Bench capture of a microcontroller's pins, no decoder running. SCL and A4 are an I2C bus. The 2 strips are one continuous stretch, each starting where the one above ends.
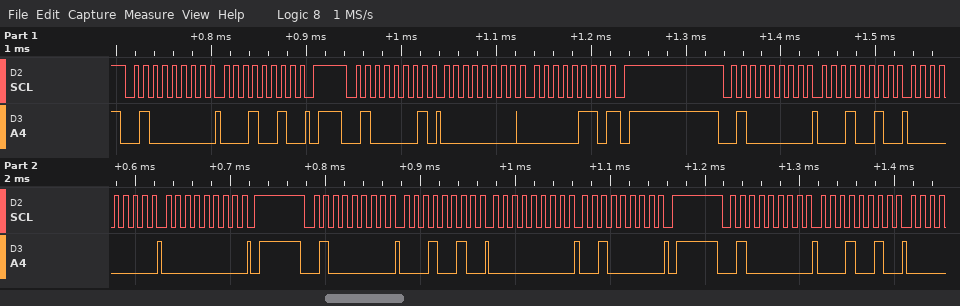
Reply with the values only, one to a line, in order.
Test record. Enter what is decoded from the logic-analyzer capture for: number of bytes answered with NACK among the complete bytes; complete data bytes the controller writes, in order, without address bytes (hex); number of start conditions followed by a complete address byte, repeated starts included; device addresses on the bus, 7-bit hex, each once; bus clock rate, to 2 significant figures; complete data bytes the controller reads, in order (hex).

1
12 12 00 00 12 00 20 12
5
0x20
100 kHz
00 06
